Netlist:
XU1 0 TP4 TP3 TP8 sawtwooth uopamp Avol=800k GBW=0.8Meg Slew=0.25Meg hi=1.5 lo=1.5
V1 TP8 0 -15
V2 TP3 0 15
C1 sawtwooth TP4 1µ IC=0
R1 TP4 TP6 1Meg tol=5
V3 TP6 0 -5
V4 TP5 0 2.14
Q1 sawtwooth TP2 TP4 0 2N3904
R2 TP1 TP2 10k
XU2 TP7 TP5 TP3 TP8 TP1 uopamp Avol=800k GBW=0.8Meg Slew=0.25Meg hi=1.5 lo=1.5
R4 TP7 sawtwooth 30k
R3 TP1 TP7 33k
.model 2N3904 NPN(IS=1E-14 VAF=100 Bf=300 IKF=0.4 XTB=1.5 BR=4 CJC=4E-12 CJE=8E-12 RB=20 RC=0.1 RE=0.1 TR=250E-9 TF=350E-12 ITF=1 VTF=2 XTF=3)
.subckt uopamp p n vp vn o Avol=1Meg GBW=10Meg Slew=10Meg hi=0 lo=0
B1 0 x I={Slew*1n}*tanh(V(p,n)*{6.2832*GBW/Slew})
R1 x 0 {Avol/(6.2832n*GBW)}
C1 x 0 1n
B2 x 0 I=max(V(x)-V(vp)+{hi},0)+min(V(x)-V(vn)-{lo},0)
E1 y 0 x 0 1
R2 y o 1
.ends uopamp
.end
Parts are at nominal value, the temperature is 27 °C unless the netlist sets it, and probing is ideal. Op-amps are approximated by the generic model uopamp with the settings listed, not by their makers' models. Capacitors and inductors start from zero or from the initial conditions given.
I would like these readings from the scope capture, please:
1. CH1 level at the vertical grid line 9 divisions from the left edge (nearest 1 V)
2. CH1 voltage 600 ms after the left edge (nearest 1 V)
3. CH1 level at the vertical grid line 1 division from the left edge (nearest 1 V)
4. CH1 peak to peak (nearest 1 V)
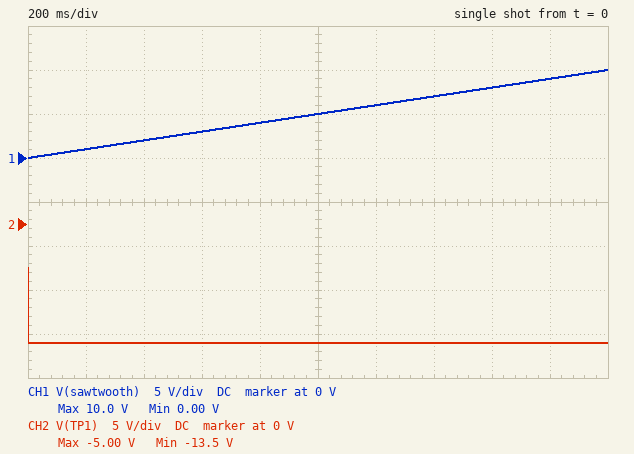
9 V
3 V
1 V
10 V
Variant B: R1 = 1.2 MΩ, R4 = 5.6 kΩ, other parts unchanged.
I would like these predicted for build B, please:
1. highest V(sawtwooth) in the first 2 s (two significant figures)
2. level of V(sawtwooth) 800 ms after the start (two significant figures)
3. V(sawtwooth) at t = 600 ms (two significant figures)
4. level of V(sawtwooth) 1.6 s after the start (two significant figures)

4.8 V
3.3 V
2.5 V
1.9 V
